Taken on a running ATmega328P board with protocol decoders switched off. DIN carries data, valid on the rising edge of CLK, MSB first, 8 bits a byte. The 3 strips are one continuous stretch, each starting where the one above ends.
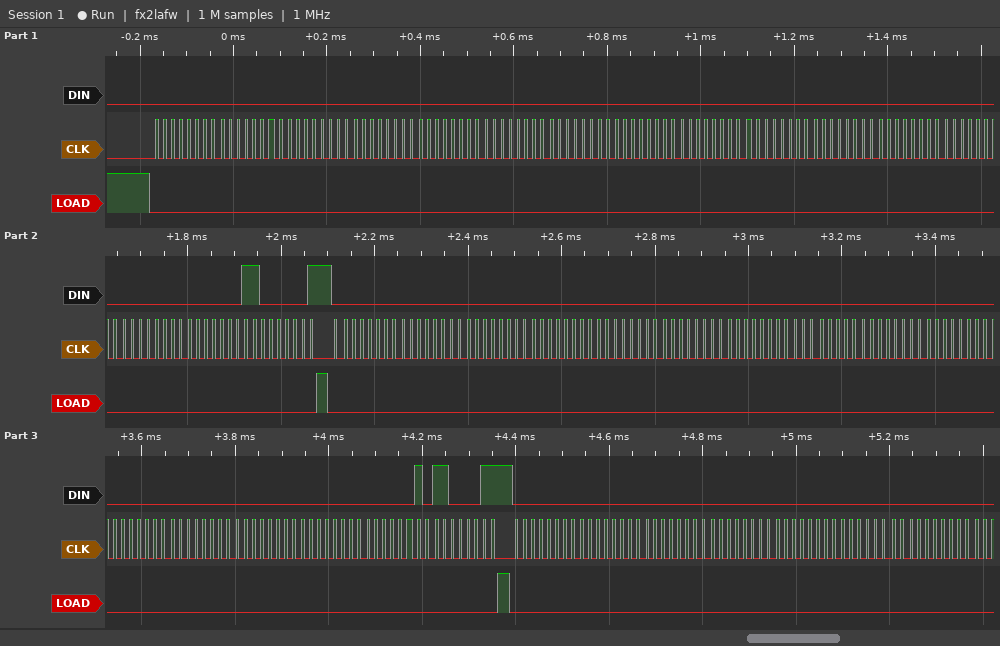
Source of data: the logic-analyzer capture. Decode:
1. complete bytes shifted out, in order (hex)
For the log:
0x00 0x00 0x00 0x00 0x00 0x00 0x00 0x00 0x00 0x00 0x00 0x00 0x00 0x00 0x01 0x81 0x00 0x00 0x00 0x00 0x00 0x00 0x00 0x00 0x00 0x00 0x00 0x00 0x00 0x00 0x02 0xC3 0x00 0x00 0x00 0x00 0x00 0x00 0x00
